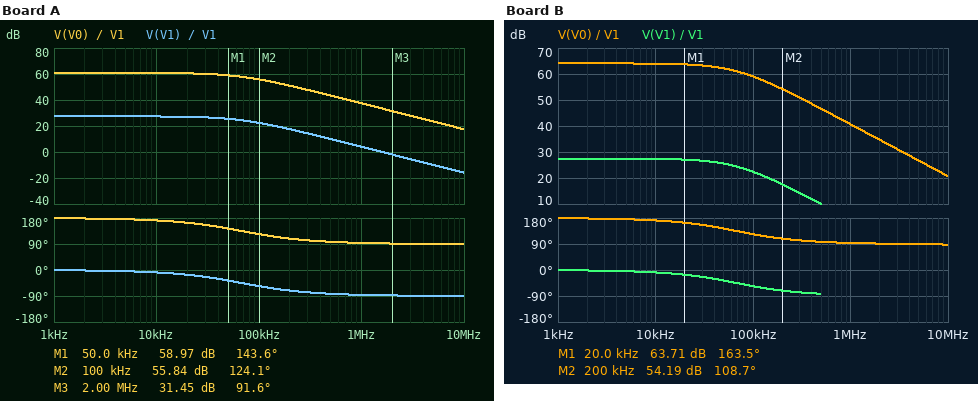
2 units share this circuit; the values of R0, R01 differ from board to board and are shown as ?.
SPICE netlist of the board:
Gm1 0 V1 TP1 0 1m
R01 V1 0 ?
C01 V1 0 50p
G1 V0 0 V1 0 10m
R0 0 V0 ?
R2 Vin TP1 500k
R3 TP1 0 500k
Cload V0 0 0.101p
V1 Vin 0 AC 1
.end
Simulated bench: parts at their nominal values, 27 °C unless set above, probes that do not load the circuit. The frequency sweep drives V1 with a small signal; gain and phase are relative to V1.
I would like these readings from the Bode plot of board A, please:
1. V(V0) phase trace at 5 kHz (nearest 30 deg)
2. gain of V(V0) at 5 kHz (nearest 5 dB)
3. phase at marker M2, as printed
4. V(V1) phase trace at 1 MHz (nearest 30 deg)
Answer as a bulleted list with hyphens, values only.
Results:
- 180 deg
- 60 dB
- 124.1 deg
- -90 deg
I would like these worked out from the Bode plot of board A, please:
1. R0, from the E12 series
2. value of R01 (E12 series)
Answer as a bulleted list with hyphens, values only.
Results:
- 4.7 kΩ
- 47 kΩ
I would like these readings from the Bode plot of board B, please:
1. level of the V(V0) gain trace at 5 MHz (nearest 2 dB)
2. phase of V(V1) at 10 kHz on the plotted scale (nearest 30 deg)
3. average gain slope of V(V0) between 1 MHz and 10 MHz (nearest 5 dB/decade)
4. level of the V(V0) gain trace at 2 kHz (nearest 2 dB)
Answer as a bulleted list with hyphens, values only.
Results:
- 26 dB
- 0 deg
- -20 dB/decade
- 64 dB
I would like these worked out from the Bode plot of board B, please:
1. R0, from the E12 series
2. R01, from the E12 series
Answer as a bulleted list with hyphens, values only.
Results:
- 6.8 kΩ
- 47 kΩ
